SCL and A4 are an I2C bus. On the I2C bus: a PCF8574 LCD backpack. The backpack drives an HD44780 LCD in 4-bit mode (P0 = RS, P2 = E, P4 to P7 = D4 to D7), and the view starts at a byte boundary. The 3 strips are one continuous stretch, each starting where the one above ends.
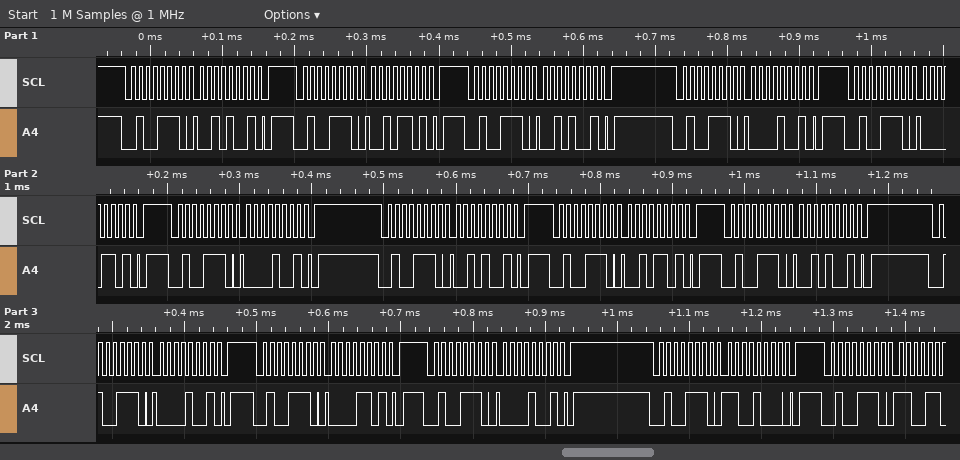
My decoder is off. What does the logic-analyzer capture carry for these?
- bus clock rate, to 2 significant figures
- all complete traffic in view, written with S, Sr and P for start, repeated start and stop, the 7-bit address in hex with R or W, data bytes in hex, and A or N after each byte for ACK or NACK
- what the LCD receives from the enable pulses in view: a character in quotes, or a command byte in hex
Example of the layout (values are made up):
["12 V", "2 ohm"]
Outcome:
["100 kHz", "S 27W A 29 A P S 27W A 2D A P S 27W A 29 A P S 27W A 09 A P S 27W A 0D A P S 27W A 09 A P S 27W A 29 A P S 27W A 2D A P S 27W A 29 A P S 27W A 09 A P S 27W A 0D A P S 27W A 09 A P S 27W A C8 A P S 27W A", "' ' ' '"]
